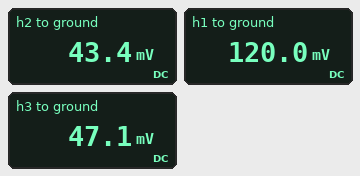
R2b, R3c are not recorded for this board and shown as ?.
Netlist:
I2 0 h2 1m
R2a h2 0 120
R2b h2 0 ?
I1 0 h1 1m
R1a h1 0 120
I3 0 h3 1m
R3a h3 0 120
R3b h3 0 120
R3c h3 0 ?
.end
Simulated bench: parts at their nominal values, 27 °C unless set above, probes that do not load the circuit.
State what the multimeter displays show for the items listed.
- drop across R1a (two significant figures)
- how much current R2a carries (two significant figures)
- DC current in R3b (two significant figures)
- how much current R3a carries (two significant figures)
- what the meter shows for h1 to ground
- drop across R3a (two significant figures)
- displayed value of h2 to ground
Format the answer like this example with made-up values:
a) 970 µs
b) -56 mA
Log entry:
a) 120 mV
b) 360 µA
c) 390 µA
d) 390 µA
e) 120.0 mV
f) 47 mV
g) 43.4 mV
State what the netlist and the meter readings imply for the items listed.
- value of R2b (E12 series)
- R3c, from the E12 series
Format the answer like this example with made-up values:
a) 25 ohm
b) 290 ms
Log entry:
a) 68 Ω
b) 220 Ω
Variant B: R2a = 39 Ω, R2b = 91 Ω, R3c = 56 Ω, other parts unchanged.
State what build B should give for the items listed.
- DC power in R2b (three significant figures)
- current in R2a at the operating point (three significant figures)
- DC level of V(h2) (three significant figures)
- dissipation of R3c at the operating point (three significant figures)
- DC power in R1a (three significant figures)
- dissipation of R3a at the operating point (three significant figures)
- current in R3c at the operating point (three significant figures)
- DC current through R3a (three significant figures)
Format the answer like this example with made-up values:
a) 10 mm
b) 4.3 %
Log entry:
a) 8.19 µW
b) 700 µA
c) 27.3 mV
d) 15.0 µW
e) 120 µW
f) 6.99 µW
g) 517 µA
h) 241 µA
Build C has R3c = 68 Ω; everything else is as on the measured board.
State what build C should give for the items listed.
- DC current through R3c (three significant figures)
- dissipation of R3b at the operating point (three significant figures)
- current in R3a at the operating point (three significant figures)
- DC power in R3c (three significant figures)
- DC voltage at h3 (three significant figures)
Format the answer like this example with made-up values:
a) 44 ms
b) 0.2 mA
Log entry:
a) 469 µA
b) 8.47 µW
c) 266 µA
d) 14.9 µW
e) 31.9 mV
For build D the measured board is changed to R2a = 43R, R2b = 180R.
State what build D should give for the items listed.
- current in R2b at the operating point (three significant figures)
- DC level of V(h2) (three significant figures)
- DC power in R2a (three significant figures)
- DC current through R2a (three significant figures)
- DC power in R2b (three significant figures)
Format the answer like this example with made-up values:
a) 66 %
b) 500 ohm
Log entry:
a) 193 µA
b) 34.7 mV
c) 28.0 µW
d) 807 µA
e) 6.69 µW
